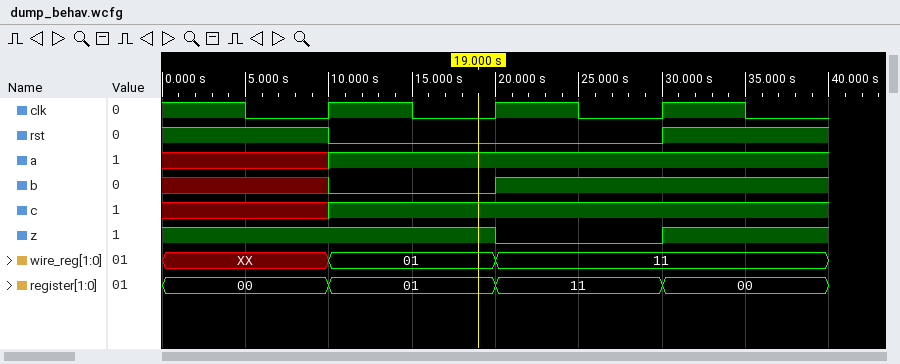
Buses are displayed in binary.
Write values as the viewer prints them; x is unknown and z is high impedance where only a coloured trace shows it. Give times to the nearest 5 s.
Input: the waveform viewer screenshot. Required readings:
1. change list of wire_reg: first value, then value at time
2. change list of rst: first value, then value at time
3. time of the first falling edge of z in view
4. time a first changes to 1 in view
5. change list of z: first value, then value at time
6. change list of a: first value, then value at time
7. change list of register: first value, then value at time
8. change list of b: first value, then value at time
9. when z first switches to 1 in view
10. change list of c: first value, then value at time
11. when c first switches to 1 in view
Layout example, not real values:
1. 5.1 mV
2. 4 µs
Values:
1. XX, 01 at 10 s, 11 at 20 s
2. 1, 0 at 10 s, 1 at 30 s
3. 20 s
4. 10 s
5. 1, 0 at 20 s, 1 at 30 s
6. x, 1 at 10 s
7. 00, 01 at 10 s, 11 at 20 s, 00 at 30 s
8. x, 0 at 10 s, 1 at 20 s
9. 30 s
10. x, 1 at 10 s
11. 10 s
